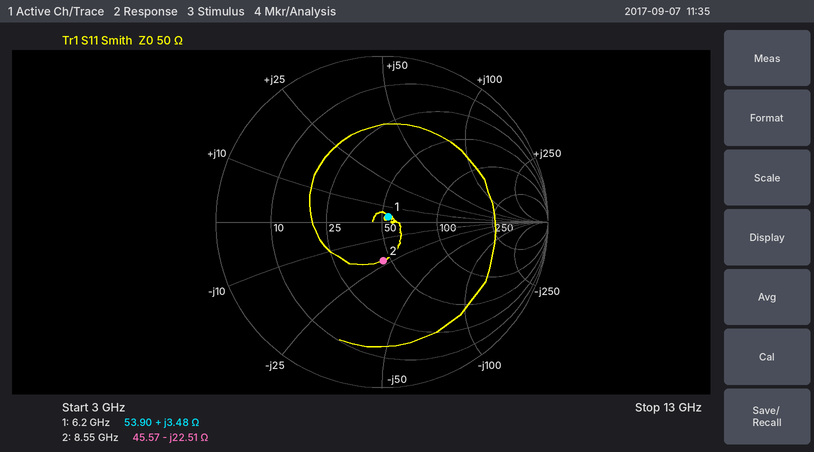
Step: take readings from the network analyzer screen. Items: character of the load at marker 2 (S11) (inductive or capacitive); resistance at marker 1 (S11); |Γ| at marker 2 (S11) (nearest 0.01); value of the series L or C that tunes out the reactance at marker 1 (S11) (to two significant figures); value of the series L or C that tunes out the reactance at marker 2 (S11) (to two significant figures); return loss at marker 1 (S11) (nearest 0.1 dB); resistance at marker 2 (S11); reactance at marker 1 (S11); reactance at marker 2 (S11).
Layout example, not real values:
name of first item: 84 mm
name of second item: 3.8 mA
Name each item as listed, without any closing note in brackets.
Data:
character of the load at marker 2 (S11): capacitive
resistance at marker 1: 53.90 Ω
|Γ| at marker 2 (S11): 0.23
value of the series L or C that tunes out the reactance at marker 1 (S11): 7.4 pF
value of the series L or C that tunes out the reactance at marker 2 (S11): 420 pH
return loss at marker 1 (S11): 26.0 dB
resistance at marker 2: 45.57 Ω
reactance at marker 1: +3.48 Ω
reactance at marker 2: -22.51 Ω
